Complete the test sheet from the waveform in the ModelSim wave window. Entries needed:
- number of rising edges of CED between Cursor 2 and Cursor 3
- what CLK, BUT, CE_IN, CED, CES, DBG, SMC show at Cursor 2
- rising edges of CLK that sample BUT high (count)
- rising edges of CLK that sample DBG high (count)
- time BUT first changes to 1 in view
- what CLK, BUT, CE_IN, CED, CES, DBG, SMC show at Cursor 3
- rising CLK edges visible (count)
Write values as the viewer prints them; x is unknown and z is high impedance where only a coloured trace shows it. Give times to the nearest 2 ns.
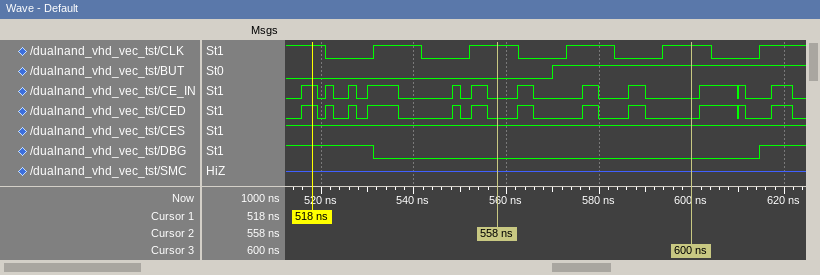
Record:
3
CLK=1, BUT=0, CE_IN=0, CED=0, CES=1, DBG=0, SMC=z
3
1
570 ns
CLK=1, BUT=1, CE_IN=0, CED=0, CES=1, DBG=0, SMC=z
5
